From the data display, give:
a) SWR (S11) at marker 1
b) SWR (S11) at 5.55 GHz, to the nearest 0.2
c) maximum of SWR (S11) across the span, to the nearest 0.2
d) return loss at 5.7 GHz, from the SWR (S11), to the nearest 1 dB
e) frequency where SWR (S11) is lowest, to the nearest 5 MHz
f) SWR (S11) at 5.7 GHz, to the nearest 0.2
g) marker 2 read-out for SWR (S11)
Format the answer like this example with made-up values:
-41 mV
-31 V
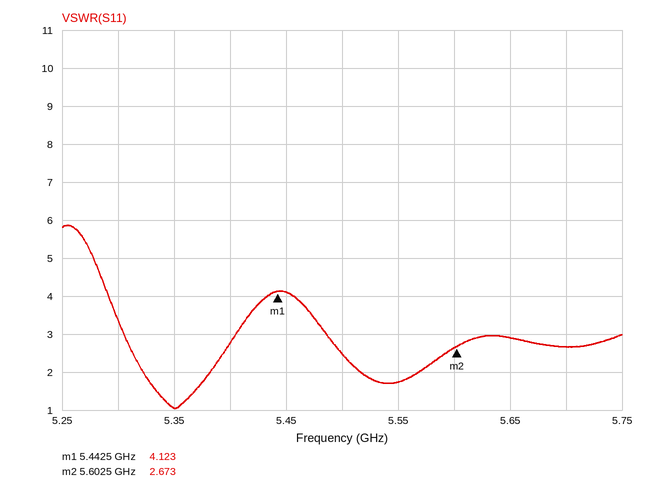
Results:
4.123
1.8
5.8
7 dB
5.350 GHz
2.6
2.673
